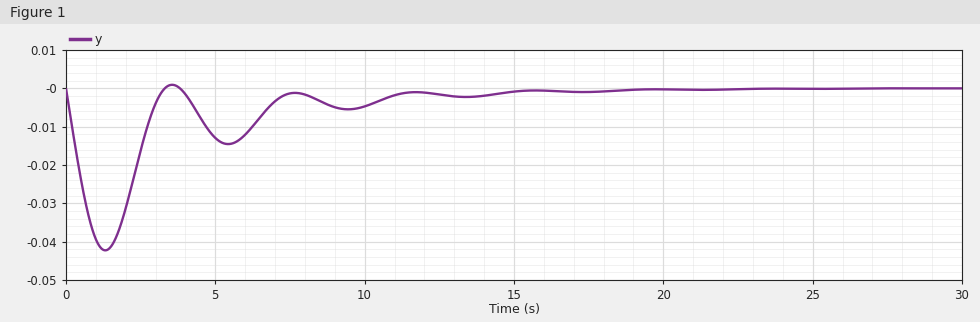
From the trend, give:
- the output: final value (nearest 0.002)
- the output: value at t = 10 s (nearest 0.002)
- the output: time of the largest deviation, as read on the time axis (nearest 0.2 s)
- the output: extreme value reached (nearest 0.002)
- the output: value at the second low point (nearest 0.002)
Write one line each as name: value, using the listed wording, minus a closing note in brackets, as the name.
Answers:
the output: final value: 0.000
the output: value at t = 10 s: -0.004
the output: time of the largest deviation, as read on the time axis: 1.4 s
the output: extreme value reached: -0.042
the output: value at the second low point: -0.014
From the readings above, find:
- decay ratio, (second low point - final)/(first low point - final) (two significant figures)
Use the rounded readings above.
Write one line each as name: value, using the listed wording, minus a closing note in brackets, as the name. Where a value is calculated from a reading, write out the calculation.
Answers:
decay ratio, (second low point - final)/(first low point - final): (-0.014 - 0) / (-0.042 - 0) = 0.33
